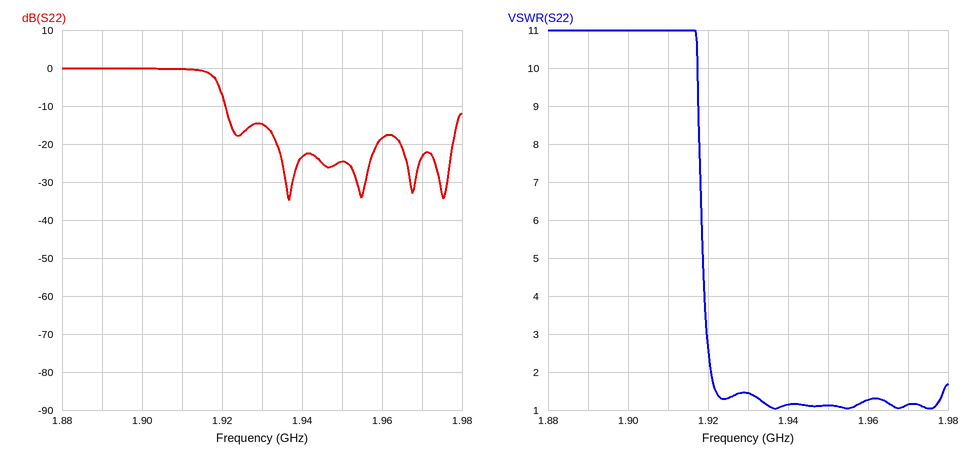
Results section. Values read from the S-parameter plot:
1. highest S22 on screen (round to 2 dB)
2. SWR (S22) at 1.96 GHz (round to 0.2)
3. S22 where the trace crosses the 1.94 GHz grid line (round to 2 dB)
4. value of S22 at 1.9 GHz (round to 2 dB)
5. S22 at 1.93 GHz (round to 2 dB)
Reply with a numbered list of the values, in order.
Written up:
1. 0 dB
2. 1.2
3. -24 dB
4. 0 dB
5. -14 dB
